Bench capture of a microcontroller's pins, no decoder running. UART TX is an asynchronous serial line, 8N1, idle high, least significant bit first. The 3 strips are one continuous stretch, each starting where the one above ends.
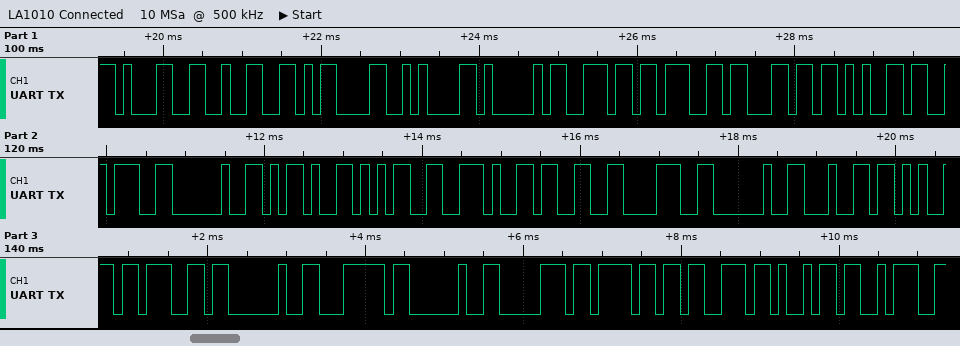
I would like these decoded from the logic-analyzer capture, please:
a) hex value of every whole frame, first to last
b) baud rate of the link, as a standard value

0x31 0x32 0x0D 0x0A 0x41 0x6E 0x67 0x6C 0x65 0x3A 0x20 0x2D 0x35 0x2E 0x33 0x38 0x20 0x64 0x65 0x67 0x20 0x7C 0x20 0x70 0x6F 0x73 0x69 0x3A
9600 baud
